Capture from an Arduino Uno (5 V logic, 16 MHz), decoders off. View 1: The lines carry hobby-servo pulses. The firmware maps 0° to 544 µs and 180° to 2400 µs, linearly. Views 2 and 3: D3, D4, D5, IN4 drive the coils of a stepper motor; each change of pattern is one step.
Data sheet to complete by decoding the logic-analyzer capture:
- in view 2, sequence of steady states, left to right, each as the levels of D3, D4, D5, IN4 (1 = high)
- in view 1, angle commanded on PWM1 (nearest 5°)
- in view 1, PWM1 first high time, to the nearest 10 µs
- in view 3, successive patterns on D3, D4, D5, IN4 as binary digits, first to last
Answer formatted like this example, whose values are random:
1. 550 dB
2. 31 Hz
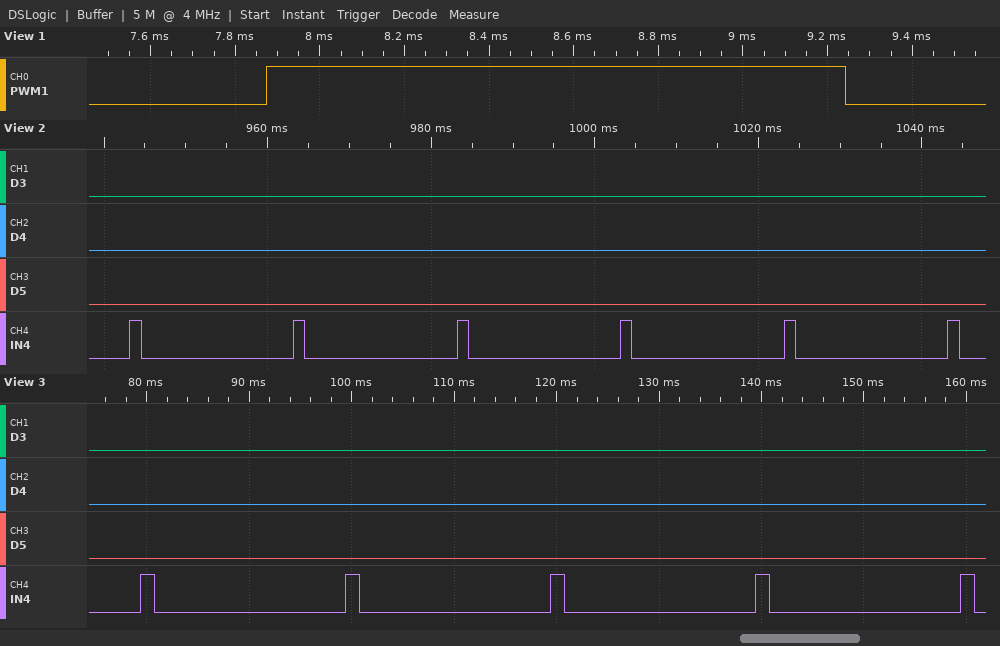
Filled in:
1. 0000 0001 0000 0001 0000 0001 0000 0001 0000 0001 0000 0001 0000
2. 80°
3. 1370 µs
4. 0000 0001 0000 0001 0000 0001 0000 0001 0000 0001 0000
